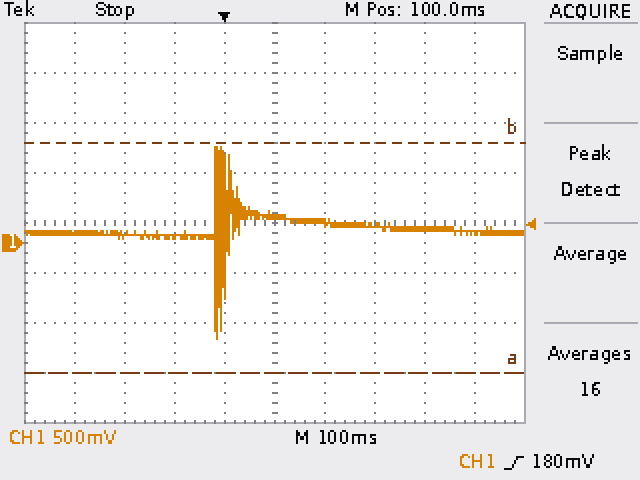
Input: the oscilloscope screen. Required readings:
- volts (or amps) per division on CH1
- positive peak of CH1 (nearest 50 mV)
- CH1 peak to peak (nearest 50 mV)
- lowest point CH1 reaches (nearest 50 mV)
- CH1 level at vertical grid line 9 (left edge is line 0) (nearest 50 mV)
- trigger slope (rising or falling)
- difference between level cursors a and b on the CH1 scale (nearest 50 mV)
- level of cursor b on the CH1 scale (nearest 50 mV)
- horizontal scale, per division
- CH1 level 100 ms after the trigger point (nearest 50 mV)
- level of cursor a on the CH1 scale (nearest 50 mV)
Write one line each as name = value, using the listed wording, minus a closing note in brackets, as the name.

volts (or amps) per division on CH1 = 500 mV
positive peak of CH1 = 950 mV
CH1 peak to peak = 1.90 V
lowest point CH1 reaches = -950 mV
CH1 level at vertical grid line 9 (left edge is line 0) = 100 mV
trigger slope = rising
difference between level cursors a and b on the CH1 scale = 2.30 V
level of cursor b on the CH1 scale = 1.00 V
horizontal scale, per division = 100 ms
CH1 level 100 ms after the trigger point = 250 mV
level of cursor a on the CH1 scale = -1.30 V
